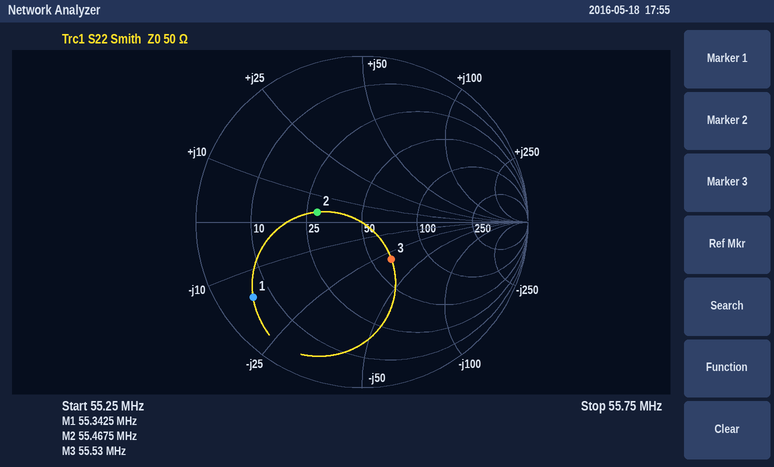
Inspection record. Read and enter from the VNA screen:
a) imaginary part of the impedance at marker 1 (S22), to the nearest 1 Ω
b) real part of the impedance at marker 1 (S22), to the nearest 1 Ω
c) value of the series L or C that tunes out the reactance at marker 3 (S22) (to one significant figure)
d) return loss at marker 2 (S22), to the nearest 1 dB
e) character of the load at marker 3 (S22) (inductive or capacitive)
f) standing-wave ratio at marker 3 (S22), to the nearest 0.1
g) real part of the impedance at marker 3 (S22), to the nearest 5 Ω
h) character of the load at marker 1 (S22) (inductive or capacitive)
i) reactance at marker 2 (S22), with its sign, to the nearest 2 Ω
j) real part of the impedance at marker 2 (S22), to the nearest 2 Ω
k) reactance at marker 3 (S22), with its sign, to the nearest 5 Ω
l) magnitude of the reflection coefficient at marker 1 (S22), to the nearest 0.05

-15 Ω
6 Ω
90 nH
11 dB
capacitive
1.8
65 Ω
capacitive
+4 Ω
28 Ω
-30 Ω
0.80
